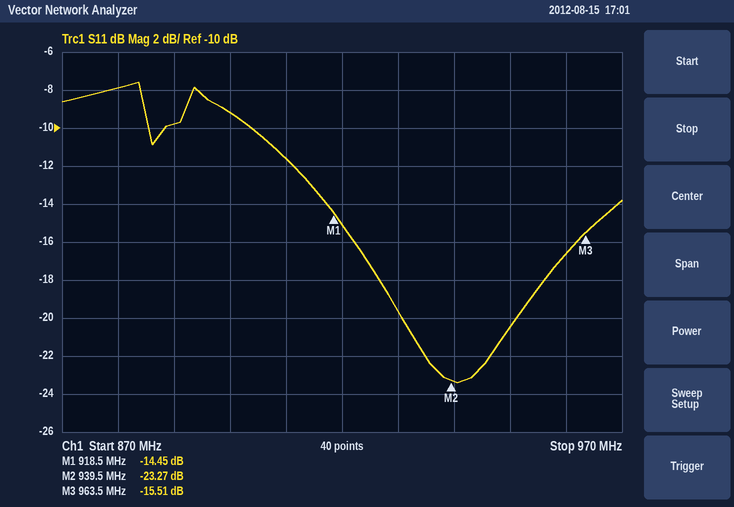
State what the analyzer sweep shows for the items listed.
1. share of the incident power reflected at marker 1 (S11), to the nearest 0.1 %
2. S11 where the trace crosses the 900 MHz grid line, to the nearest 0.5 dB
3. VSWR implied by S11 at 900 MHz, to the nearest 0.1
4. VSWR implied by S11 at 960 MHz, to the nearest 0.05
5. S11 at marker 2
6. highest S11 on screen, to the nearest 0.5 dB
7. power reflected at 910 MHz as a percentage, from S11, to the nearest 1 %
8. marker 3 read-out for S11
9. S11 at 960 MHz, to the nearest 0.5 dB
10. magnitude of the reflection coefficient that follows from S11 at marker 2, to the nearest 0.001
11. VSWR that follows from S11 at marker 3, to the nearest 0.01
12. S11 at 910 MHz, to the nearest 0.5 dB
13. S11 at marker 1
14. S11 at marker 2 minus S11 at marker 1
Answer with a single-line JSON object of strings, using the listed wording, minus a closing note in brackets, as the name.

{"share of the incident power reflected at marker 1 (S11), to the nearest 0.1 %": "3.6 %", "S11 where the trace crosses the 900 MHz grid line, to the nearest 0.5 dB": "-9.0 dB", "VSWR implied by S11 at 900 MHz, to the nearest 0.1": "2.1", "VSWR implied by S11 at 960 MHz, to the nearest 0.05": "1.35", "S11 at marker 2": "-23.27 dB", "highest S11 on screen, to the nearest 0.5 dB": "-7.5 dB", "power reflected at 910 MHz as a percentage, from S11, to the nearest 1 %": "7 %", "marker 3 read-out for S11": "-15.51 dB", "S11 at 960 MHz, to the nearest 0.5 dB": "-16.5 dB", "magnitude of the reflection coefficient that follows from S11 at marker 2, to the nearest 0.001": "0.069", "VSWR that follows from S11 at marker 3, to the nearest 0.01": "1.40", "S11 at 910 MHz, to the nearest 0.5 dB": "-11.5 dB", "S11 at marker 1": "-14.45 dB", "S11 at marker 2 minus S11 at marker 1": "-8.82 dB"}
